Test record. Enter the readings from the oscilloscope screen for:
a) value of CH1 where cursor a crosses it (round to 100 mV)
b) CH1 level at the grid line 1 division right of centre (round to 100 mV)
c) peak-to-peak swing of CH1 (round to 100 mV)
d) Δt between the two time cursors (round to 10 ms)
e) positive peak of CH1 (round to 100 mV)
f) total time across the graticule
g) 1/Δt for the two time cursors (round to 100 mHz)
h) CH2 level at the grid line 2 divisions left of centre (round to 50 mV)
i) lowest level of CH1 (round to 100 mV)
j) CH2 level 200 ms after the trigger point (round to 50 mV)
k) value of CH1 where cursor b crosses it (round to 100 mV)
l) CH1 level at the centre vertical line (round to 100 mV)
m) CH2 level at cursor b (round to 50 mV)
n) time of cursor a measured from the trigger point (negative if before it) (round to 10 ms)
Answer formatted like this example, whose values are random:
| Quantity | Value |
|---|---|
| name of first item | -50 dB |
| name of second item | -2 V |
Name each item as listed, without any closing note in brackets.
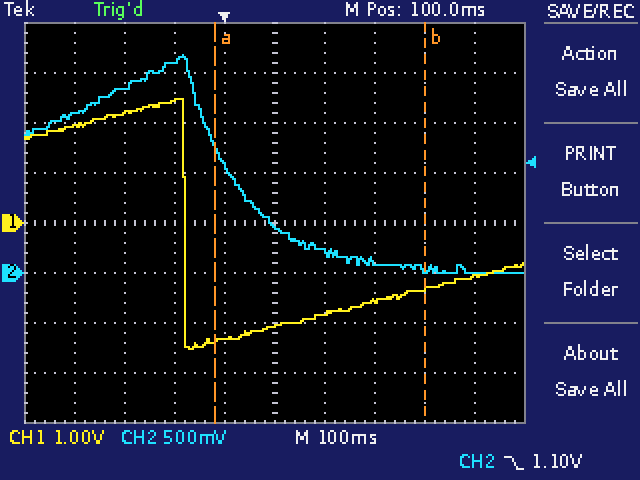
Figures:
| Quantity | Value |
|---|---|
| value of CH1 where cursor a crosses it | -2.4 V |
| CH1 level at the grid line 1 division right of centre | -1.8 V |
| peak-to-peak swing of CH1 | 5.0 V |
| Δt between the two time cursors | 420 ms |
| positive peak of CH1 | 2.5 V |
| total time across the graticule | 1 s |
| 1/Δt for the two time cursors | 2.4 Hz |
| CH2 level at the grid line 2 divisions left of centre | 2.10 V |
| lowest level of CH1 | -2.5 V |
| CH2 level 200 ms after the trigger point | 200 mV |
| value of CH1 where cursor b crosses it | -1.3 V |
| CH1 level at the centre vertical line | -2.1 V |
| CH2 level at cursor b | 50 mV |
| time of cursor a measured from the trigger point (negative if before it) | -20 ms |
